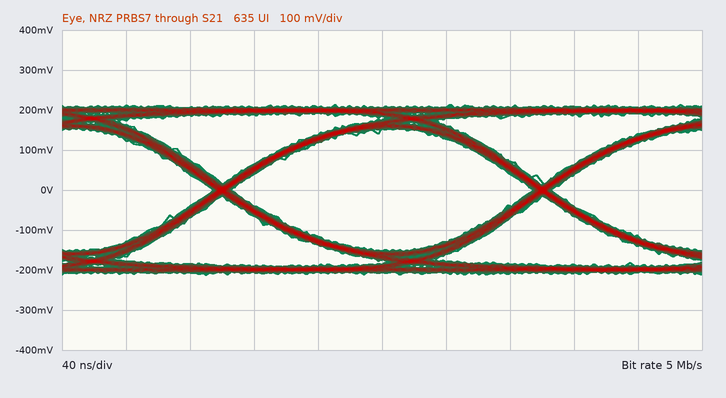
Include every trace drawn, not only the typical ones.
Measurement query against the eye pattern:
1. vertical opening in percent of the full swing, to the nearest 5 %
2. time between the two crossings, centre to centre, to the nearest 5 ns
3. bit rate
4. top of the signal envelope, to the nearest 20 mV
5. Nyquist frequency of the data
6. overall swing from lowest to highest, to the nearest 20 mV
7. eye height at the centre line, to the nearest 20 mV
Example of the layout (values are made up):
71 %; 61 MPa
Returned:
70 %; 200 ns; 5 Mb/s; 220 mV; 2.5 MHz; 420 mV; 300 mV
